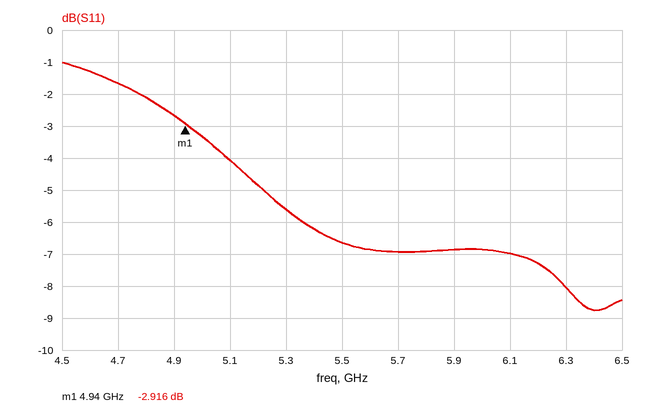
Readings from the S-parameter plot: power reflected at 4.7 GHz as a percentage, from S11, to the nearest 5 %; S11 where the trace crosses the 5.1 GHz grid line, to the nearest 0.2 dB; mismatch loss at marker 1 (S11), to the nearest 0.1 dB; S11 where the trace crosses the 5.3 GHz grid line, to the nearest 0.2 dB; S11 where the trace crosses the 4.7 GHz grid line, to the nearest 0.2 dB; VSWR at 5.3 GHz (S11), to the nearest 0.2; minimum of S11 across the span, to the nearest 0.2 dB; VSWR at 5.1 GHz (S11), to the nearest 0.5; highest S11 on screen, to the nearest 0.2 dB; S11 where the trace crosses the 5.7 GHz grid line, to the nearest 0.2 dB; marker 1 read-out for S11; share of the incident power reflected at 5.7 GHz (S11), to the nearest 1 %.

70 %
-4.0 dB
3.1 dB
-5.6 dB
-1.6 dB
3.2
-8.8 dB
4.5
-1.0 dB
-7.0 dB
-2.916 dB
20 %
